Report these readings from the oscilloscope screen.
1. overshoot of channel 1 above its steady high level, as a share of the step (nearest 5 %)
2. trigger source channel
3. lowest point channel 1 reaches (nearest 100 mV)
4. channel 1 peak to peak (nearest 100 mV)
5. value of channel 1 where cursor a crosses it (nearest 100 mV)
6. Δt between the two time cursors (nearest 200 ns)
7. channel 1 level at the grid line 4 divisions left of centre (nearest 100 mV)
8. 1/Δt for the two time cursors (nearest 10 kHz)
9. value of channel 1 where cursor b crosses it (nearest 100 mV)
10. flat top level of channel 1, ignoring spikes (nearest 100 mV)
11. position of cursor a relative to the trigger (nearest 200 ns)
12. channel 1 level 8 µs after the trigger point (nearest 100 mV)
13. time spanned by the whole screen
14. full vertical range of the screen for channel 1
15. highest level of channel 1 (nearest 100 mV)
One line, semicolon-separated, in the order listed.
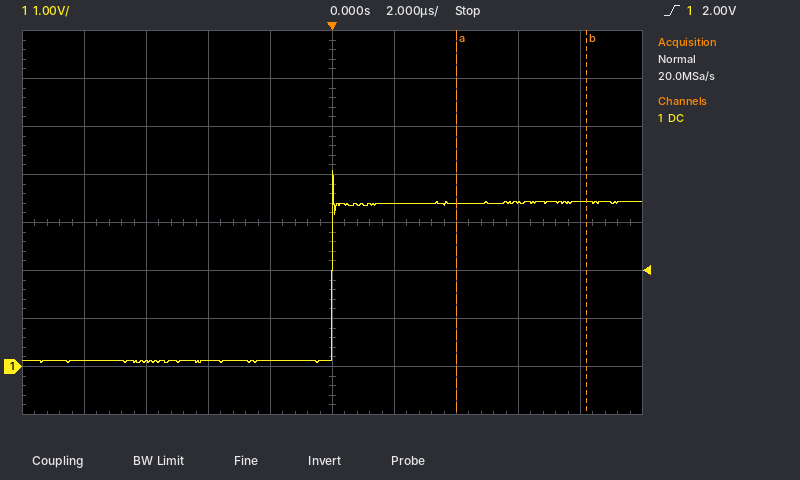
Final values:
20 %; channel 1; 100 mV; 4.0 V; 3.4 V; 4.2 µs; 100 mV; 240 kHz; 3.4 V; 3.4 V; +4.0 µs; 3.4 V; 20 µs; 8 V; 4.1 V
